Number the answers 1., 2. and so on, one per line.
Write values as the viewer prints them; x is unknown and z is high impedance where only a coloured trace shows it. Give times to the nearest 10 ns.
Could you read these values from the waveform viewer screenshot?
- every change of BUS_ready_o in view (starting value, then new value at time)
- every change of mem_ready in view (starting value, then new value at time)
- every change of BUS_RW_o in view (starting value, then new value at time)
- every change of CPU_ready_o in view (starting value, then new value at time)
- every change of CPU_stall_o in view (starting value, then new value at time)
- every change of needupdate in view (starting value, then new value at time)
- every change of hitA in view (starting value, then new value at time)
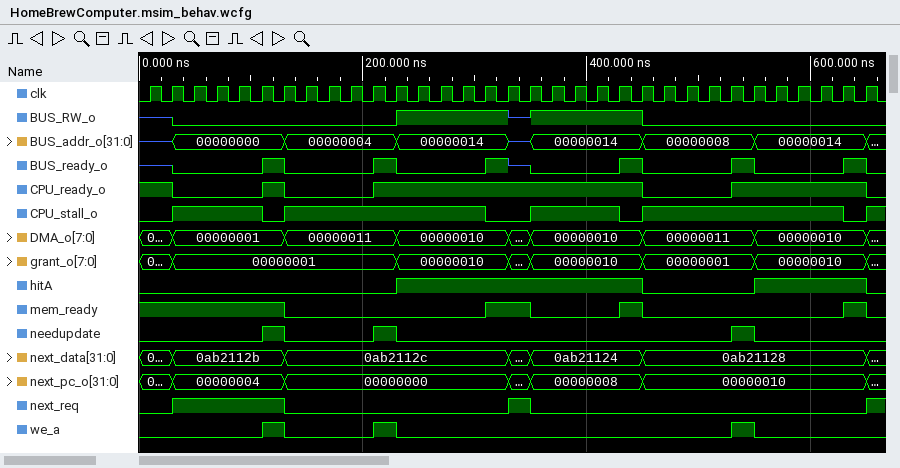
1. z, 0 at 30 ns, 1 at 110 ns, 0 at 130 ns, 1 at 210 ns, 0 at 230 ns, 1 at 310 ns, z at 330 ns, 0 at 350 ns, 1 at 430 ns, 0 at 450 ns, 1 at 530 ns, 0 at 550 ns, 1 at 630 ns, 0 at 650 ns
2. 1, 0 at 130 ns, 1 at 310 ns, 0 at 350 ns, 1 at 430 ns, 0 at 450 ns, 1 at 630 ns, 0 at 650 ns
3. z, 0 at 30 ns, 1 at 230 ns, z at 330 ns, 1 at 350 ns, 0 at 450 ns
4. 1, 0 at 30 ns, 1 at 110 ns, 0 at 130 ns, 1 at 210 ns, 0 at 450 ns, 1 at 530 ns, 0 at 650 ns
5. 0, 1 at 30 ns, 0 at 110 ns, 1 at 130 ns, 0 at 310 ns, 1 at 350 ns, 0 at 430 ns, 1 at 450 ns, 0 at 630 ns, 1 at 650 ns
6. 0, 1 at 110 ns, 0 at 130 ns, 1 at 210 ns, 0 at 230 ns, 1 at 530 ns, 0 at 550 ns
7. 0, 1 at 230 ns, 0 at 450 ns, 1 at 550 ns, 0 at 650 ns
